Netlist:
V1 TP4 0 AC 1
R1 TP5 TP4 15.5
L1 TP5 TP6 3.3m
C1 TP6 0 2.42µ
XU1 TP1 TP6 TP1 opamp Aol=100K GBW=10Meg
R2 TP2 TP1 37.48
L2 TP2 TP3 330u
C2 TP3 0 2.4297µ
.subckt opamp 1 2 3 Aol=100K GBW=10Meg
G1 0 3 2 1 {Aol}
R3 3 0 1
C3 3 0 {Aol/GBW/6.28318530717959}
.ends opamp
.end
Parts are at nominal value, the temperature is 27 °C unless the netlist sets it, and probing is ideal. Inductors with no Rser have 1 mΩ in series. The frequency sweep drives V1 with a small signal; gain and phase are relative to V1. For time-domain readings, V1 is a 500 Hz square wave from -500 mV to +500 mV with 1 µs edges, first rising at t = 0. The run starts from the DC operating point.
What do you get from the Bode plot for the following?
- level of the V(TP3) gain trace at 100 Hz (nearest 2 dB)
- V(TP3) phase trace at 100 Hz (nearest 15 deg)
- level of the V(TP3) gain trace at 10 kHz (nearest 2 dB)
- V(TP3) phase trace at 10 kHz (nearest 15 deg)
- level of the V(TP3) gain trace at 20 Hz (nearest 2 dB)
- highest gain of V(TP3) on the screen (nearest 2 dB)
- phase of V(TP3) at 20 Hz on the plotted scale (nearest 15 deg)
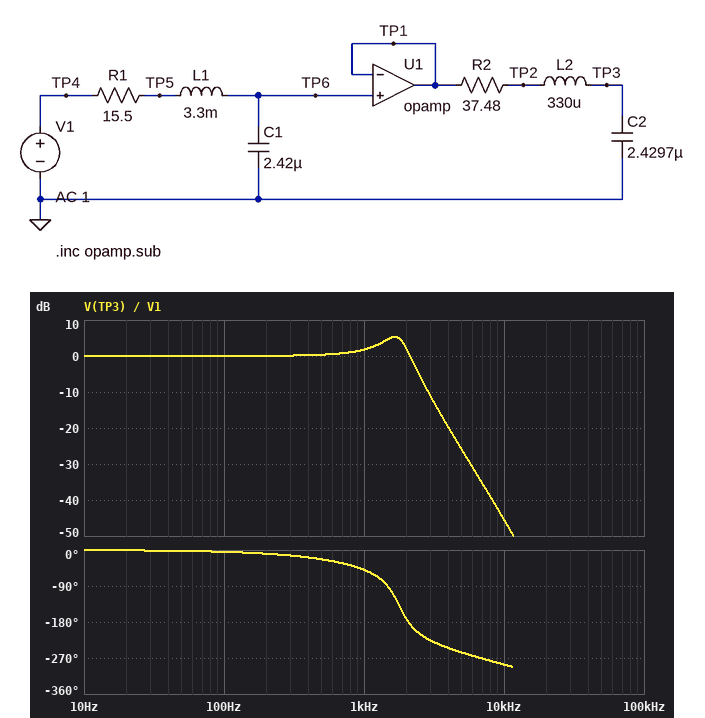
0 dB
0 deg
-46 dB
-285 deg
0 dB
6 dB
0 deg
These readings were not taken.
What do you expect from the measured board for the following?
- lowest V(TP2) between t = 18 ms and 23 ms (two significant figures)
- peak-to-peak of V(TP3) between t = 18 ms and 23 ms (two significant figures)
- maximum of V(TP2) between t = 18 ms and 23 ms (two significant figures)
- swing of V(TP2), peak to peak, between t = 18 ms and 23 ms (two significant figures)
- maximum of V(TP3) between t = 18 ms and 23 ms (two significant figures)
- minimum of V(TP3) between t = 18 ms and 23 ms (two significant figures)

-820 mV
1.7 V
820 mV
1.6 V
850 mV
-850 mV
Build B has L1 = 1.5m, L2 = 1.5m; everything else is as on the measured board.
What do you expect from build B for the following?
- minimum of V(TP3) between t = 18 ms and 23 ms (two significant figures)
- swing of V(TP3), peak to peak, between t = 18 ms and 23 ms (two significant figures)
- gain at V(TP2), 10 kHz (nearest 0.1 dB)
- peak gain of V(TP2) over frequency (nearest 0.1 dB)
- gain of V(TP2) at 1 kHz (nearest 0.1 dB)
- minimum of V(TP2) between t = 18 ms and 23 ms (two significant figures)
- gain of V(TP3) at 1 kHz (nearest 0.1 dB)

-750 mV
1.5 V
-23.4 dB
0 dB
-0.6 dB
-610 mV
0.8 dB
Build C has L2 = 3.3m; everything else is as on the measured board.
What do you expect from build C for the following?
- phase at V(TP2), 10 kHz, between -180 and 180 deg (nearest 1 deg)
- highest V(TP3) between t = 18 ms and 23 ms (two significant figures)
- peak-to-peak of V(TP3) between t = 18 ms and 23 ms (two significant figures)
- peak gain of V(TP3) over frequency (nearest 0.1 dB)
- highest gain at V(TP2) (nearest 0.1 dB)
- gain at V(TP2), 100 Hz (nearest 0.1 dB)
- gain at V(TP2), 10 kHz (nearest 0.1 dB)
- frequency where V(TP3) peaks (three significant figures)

-165 deg
1.1 V
2.2 V
8.1 dB
0.5 dB
0 dB
-29.9 dB
1.63 kHz
